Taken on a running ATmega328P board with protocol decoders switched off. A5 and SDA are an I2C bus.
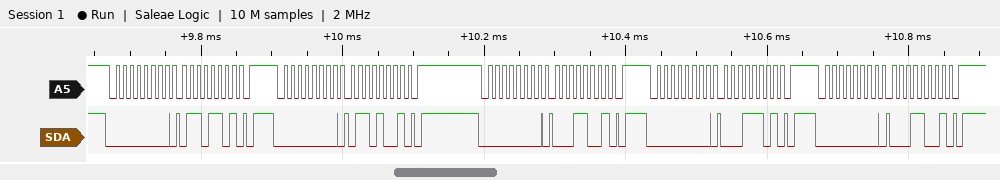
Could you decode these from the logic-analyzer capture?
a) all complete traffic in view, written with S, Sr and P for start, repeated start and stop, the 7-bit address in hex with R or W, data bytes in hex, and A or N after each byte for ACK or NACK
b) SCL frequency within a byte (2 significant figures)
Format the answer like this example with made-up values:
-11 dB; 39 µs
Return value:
S 00W A 6D A P S 00W A 69 A P S 00W A 19 A P S 00W A 1D A P S 00W A 19 A P; 100 kHz
